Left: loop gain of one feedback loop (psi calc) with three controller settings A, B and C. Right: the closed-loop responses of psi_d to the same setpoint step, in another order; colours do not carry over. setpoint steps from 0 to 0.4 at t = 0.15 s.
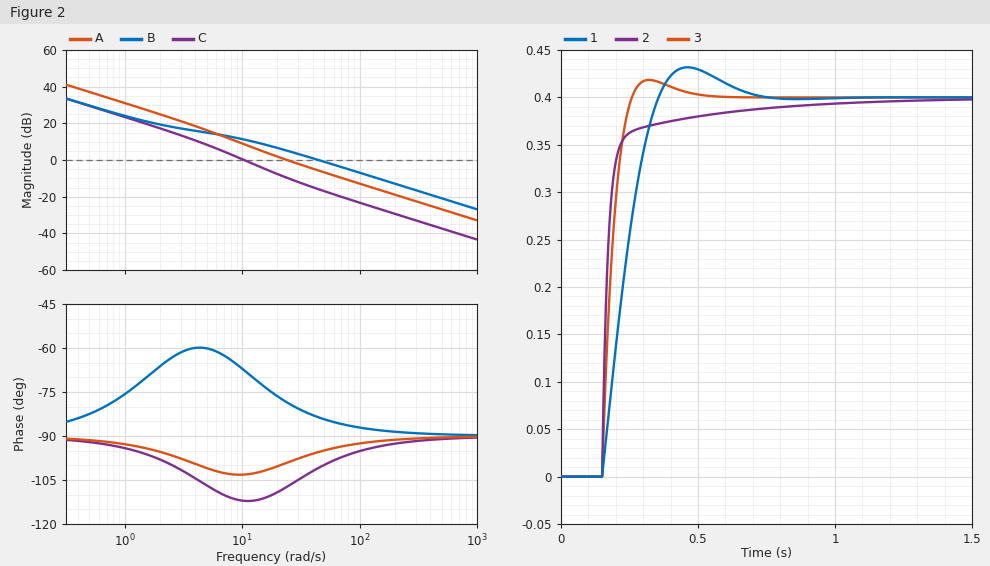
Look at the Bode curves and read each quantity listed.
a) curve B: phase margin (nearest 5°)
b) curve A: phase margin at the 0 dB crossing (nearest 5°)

95°
80°
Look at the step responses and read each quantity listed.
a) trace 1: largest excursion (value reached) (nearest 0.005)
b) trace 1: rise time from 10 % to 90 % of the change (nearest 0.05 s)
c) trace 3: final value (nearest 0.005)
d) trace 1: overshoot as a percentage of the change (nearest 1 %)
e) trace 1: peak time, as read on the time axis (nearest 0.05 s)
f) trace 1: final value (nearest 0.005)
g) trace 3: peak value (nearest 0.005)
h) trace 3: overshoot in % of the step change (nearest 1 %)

0.430
0.15 s
0.400
8 %
0.45 s
0.400
0.420
5 %
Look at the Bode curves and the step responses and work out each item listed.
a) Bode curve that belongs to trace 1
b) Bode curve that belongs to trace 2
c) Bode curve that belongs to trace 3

C
B
A
